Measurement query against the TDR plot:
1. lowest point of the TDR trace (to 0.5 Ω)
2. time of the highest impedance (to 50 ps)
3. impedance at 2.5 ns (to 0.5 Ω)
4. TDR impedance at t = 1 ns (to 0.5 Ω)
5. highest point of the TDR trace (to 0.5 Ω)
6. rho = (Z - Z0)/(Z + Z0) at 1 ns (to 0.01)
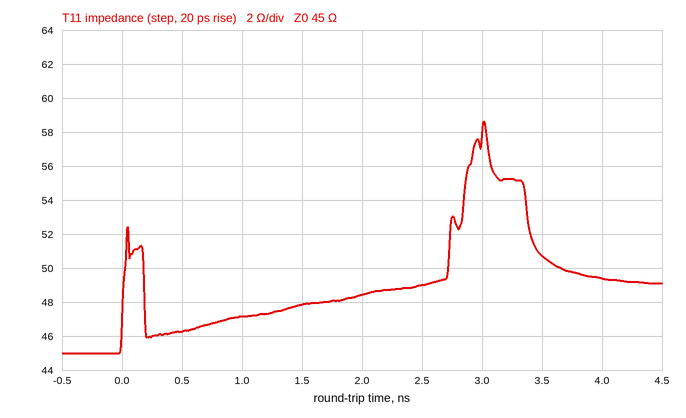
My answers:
45.0 Ω
3.00 ns
49.0 Ω
47.0 Ω
58.5 Ω
+0.02
